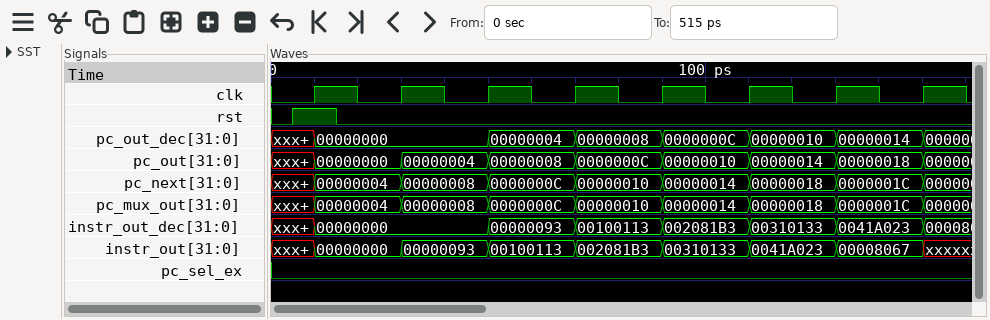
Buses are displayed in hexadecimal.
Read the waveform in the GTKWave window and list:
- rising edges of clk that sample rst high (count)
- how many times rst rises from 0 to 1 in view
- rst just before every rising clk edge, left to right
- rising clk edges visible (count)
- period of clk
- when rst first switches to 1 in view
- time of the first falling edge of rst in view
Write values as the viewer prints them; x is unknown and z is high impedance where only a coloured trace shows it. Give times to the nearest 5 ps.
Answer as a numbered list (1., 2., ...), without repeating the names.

1. 1
2. 1
3. 1 0 0 0 0 0 0 0
4. 8
5. 20 ps
6. 5 ps
7. 15 ps
